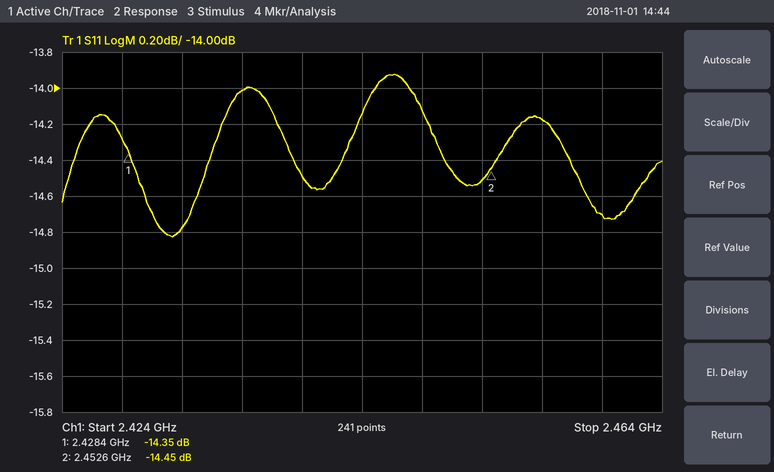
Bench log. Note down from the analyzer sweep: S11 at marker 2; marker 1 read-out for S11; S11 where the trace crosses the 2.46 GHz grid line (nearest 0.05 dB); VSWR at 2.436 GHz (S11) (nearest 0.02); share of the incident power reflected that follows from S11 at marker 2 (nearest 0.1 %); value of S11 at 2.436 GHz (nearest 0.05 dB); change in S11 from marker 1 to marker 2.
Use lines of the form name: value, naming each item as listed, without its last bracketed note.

S11 at marker 2: -14.45 dB
marker 1 read-out for S11: -14.35 dB
S11 where the trace crosses the 2.46 GHz grid line: -14.70 dB
VSWR at 2.436 GHz (S11): 1.50
share of the incident power reflected that follows from S11 at marker 2: 3.6 %
value of S11 at 2.436 GHz: -14.00 dB
change in S11 from marker 1 to marker 2: -0.10 dB
